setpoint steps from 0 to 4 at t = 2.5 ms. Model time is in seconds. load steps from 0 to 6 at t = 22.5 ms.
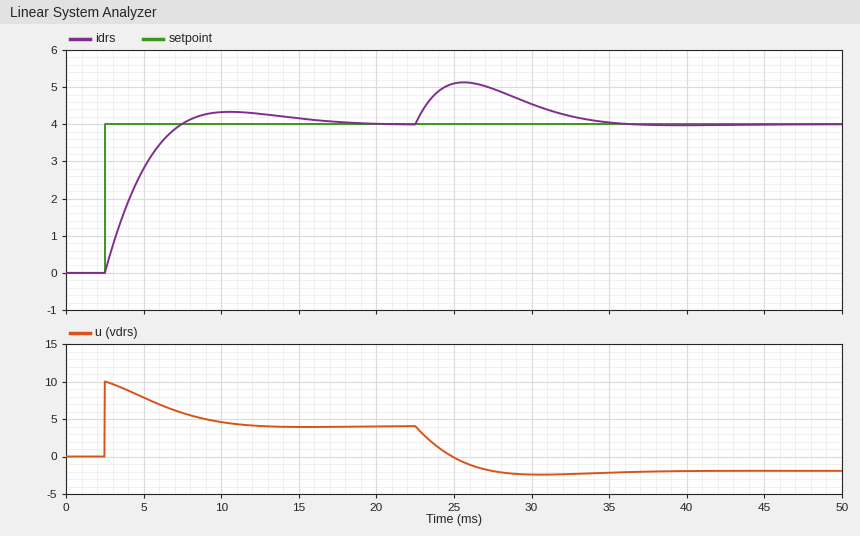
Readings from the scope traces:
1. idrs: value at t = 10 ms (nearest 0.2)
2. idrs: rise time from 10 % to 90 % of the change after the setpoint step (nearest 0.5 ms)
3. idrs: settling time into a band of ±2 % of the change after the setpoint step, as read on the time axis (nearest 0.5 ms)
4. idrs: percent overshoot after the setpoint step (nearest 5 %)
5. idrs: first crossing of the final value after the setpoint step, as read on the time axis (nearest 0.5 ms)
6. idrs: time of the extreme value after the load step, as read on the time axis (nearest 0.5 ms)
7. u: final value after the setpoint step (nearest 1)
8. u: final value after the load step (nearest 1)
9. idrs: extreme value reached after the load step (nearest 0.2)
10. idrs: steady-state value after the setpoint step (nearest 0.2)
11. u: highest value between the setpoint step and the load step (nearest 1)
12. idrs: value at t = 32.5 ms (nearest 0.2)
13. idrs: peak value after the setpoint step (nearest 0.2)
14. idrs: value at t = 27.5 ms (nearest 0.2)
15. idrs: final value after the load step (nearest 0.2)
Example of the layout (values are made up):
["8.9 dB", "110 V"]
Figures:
["4.4", "3.5 ms", "17.0 ms", "10 %", "7.5 ms", "25.5 ms", "4", "-2", "5.2", "4.0", "10", "4.2", "4.4", "5.0", "4.0"]
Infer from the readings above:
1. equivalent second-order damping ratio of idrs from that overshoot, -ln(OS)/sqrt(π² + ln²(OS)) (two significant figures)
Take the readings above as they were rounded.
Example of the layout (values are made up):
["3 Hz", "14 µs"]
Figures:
["0.59"]
